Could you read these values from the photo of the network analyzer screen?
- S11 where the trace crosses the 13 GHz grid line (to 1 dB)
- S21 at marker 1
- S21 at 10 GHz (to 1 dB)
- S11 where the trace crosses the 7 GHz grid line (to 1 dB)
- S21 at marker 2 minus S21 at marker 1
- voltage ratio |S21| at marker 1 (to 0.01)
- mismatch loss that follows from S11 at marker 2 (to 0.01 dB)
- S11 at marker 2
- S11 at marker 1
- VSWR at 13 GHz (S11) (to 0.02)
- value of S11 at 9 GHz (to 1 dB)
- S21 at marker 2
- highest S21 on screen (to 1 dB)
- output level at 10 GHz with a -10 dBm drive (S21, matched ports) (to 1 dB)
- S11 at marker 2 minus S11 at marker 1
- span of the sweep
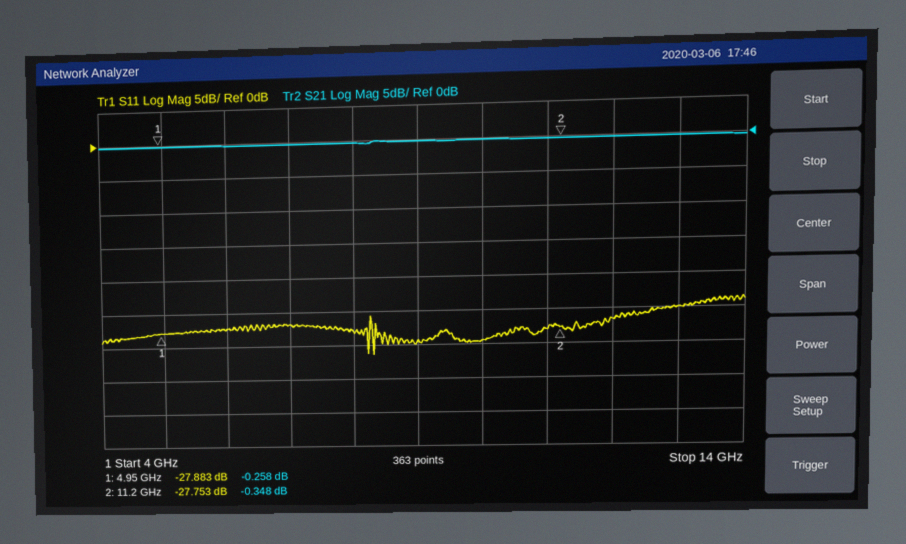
-25 dB
-0.258 dB
0 dB
-27 dB
-0.090 dB
0.97
0.01 dB
-27.753 dB
-27.883 dB
1.12
-29 dB
-0.348 dB
0 dB
-10 dBm
0.130 dB
10 GHz
